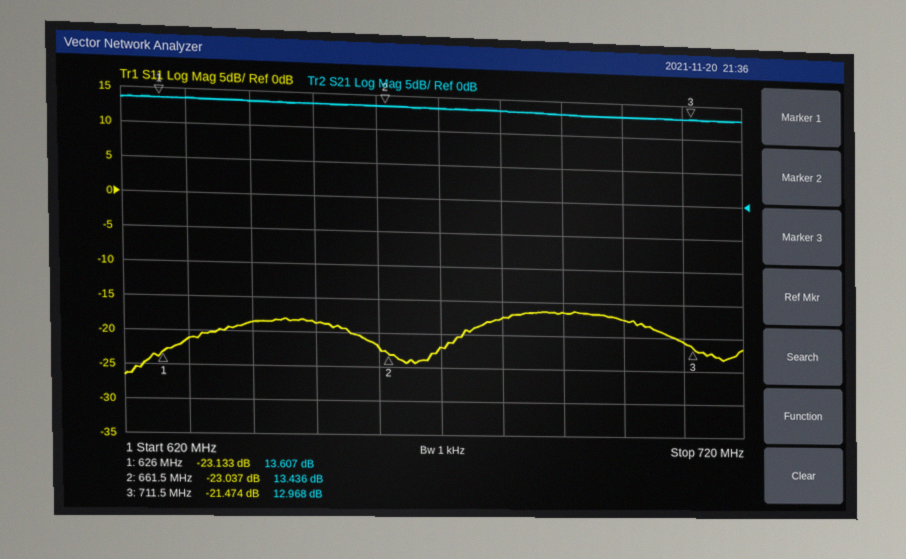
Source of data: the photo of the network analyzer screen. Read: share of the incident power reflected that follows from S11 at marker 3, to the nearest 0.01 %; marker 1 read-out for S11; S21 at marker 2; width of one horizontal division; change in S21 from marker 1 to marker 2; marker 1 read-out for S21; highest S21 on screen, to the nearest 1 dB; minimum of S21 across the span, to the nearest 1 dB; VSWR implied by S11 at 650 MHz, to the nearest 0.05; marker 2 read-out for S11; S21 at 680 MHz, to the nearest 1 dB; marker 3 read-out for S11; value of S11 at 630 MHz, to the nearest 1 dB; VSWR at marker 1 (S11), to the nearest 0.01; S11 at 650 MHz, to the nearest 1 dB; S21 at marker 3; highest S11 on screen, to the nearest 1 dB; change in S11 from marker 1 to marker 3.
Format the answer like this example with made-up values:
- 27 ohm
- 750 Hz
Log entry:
- 0.71 %
- -23.133 dB
- 13.436 dB
- 10 MHz
- -0.171 dB
- 13.607 dB
- 14 dB
- 13 dB
- 1.25
- -23.037 dB
- 13 dB
- -21.474 dB
- -21 dB
- 1.15
- -19 dB
- 12.968 dB
- -16 dB
- 1.659 dB
